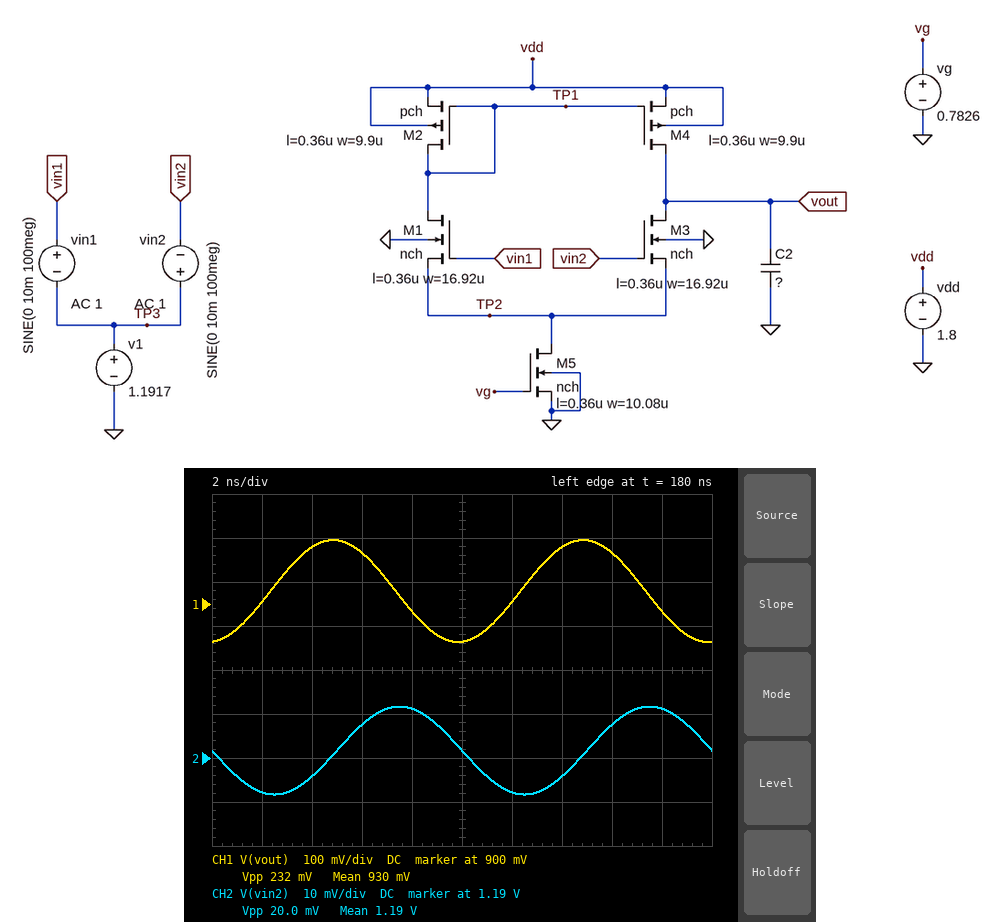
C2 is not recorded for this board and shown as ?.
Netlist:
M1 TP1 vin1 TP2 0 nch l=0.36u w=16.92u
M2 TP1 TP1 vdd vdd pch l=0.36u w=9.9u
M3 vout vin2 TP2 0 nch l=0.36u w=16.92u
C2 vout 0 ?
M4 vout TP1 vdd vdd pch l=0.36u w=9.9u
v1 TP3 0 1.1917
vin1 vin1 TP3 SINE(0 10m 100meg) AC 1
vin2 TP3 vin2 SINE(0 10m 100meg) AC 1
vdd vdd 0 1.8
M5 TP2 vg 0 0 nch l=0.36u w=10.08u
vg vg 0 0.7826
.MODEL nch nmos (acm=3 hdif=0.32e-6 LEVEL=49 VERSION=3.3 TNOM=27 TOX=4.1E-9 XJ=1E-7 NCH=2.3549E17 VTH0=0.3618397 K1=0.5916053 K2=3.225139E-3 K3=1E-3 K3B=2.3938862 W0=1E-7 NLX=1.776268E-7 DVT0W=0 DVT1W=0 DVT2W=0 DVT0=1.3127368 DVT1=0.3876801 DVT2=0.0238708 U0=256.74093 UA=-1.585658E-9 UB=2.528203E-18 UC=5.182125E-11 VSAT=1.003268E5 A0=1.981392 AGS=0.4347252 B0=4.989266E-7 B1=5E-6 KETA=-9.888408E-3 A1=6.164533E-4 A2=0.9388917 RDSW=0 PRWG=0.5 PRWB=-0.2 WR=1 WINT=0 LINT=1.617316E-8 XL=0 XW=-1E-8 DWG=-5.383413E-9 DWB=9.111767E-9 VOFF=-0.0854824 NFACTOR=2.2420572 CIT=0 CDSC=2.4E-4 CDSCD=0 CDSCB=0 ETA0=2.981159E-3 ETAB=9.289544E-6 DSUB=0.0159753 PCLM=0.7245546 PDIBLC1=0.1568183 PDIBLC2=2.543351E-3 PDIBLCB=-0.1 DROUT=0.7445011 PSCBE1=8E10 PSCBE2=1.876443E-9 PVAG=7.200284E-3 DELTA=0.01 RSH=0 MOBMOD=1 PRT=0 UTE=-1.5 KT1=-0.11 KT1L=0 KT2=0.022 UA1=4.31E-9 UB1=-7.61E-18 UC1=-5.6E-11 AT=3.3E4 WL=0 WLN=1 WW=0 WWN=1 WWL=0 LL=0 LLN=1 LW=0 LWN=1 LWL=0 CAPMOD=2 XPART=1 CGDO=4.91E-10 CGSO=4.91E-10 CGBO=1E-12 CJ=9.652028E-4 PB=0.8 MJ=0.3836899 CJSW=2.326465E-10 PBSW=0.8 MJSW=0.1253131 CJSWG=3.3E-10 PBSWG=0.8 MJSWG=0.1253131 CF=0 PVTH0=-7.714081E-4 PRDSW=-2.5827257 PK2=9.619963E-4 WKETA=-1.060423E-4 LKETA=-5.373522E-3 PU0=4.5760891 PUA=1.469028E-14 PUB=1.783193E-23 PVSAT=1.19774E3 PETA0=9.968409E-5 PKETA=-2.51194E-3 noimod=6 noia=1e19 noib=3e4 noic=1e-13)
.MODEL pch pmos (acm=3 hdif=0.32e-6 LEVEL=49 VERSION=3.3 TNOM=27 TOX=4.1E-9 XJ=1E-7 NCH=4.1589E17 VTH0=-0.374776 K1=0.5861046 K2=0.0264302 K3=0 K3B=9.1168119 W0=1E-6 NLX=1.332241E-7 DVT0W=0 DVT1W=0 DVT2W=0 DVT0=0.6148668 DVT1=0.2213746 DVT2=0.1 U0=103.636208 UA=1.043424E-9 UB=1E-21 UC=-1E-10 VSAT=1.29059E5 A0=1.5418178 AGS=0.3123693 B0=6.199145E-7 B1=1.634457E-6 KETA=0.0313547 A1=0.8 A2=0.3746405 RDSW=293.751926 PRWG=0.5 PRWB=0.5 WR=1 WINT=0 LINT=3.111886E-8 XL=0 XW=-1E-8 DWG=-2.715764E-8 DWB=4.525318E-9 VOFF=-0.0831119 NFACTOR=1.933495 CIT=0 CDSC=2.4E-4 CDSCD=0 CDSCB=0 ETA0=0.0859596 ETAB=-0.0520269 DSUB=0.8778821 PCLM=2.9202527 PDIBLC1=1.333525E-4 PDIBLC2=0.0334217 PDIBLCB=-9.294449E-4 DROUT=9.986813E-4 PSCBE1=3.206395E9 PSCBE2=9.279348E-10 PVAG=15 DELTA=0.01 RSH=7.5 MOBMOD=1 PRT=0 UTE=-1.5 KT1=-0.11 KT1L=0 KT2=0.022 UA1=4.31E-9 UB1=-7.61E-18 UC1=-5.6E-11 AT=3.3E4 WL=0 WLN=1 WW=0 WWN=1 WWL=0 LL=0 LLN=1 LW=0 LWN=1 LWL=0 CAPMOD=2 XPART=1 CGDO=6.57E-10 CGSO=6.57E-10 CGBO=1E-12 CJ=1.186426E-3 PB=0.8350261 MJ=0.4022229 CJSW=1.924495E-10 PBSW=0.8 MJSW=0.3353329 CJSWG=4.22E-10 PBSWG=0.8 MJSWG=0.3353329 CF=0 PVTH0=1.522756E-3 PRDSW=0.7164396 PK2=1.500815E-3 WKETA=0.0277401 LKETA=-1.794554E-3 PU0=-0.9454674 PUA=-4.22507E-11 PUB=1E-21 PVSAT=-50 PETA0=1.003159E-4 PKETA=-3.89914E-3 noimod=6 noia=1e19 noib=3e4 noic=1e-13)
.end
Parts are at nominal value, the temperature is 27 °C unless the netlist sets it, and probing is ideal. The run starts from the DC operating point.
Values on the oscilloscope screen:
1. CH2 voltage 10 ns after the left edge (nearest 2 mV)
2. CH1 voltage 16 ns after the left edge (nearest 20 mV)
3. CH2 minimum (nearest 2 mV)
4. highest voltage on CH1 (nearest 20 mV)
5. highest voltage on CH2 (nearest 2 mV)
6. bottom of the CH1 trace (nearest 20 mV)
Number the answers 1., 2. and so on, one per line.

1. 1.192 V
2. 1.02 V
3. 1.182 V
4. 1.04 V
5. 1.202 V
6. 820 mV
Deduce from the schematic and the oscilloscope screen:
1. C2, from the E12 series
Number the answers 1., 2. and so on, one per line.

1. 470 fF
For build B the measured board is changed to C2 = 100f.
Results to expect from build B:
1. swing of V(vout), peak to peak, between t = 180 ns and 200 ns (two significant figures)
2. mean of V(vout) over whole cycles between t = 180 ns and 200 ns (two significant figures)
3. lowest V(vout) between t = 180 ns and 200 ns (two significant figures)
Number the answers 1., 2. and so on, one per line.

1. 700 mV
2. 960 mV
3. 610 mV
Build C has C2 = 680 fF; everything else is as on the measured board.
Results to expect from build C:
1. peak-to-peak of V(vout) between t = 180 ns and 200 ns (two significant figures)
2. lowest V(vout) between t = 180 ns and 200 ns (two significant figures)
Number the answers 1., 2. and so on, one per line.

1. 170 mV
2. 850 mV
